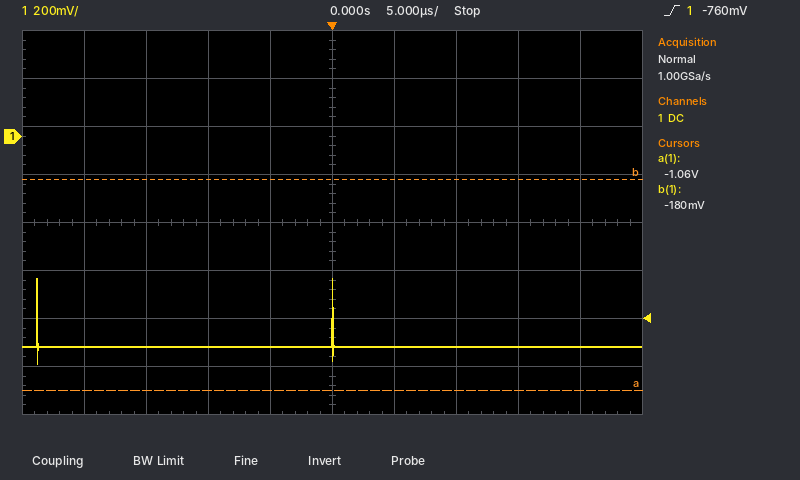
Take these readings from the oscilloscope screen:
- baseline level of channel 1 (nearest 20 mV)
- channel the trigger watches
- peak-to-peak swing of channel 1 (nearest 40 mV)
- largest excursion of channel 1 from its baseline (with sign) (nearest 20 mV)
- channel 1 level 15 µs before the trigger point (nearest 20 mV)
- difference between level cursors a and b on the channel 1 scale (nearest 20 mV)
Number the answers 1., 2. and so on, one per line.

1. -880 mV
2. channel 1
3. 360 mV
4. +280 mV
5. -880 mV
6. 880 mV
